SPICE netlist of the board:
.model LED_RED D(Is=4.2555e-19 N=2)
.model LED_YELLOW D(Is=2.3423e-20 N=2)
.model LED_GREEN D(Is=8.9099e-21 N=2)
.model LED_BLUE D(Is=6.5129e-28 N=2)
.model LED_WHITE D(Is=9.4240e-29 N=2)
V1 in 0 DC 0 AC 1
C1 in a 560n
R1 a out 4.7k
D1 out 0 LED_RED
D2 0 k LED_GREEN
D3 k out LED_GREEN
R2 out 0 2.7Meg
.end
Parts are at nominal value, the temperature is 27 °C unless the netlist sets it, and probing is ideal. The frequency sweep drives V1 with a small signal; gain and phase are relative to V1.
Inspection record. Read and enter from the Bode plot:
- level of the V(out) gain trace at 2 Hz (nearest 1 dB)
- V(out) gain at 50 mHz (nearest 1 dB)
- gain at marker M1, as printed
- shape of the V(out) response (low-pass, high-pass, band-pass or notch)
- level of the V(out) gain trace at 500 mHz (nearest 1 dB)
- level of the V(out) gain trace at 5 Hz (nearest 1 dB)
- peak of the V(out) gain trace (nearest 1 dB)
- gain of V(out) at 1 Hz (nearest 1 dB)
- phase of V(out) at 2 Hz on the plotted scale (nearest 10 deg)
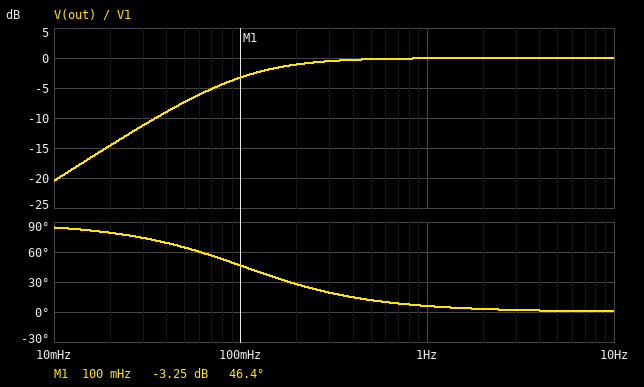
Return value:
0 dB
-7 dB
-3.25 dB
high-pass
0 dB
0 dB
0 dB
0 dB
0 deg
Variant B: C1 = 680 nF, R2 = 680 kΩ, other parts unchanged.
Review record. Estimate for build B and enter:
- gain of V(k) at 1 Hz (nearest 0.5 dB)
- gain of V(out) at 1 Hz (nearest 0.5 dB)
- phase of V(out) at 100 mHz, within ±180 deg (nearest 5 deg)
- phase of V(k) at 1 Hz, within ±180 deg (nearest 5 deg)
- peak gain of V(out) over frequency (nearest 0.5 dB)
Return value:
-6.5 dB
-0.5 dB
75 deg
20 deg
0 dB
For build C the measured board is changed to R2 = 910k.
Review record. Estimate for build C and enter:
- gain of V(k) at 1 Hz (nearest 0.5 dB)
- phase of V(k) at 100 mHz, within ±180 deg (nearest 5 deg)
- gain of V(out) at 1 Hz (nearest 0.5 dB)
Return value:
-6.5 dB
70 deg
-0.5 dB
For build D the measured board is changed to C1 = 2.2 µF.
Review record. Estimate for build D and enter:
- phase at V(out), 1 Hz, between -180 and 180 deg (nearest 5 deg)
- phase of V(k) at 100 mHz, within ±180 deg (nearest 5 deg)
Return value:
0 deg
15 deg
